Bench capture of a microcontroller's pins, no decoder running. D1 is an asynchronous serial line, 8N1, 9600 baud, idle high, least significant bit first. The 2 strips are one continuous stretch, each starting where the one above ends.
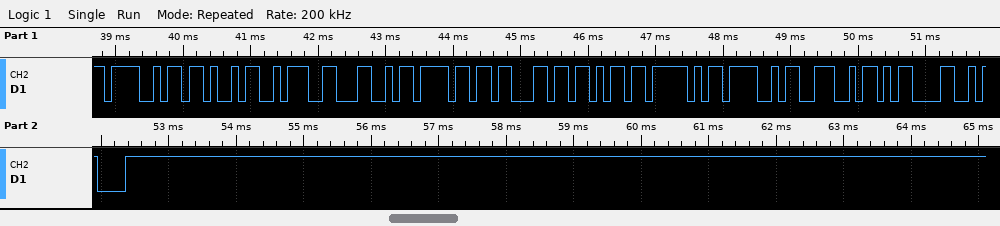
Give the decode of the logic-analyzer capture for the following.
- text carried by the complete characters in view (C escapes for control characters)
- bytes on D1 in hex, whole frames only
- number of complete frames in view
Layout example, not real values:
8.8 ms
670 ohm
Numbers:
"OK:Lock_ON\r\n"
4F 4B 3A 4C 6F 63 6B 5F 4F 4E 0D 0A
12
